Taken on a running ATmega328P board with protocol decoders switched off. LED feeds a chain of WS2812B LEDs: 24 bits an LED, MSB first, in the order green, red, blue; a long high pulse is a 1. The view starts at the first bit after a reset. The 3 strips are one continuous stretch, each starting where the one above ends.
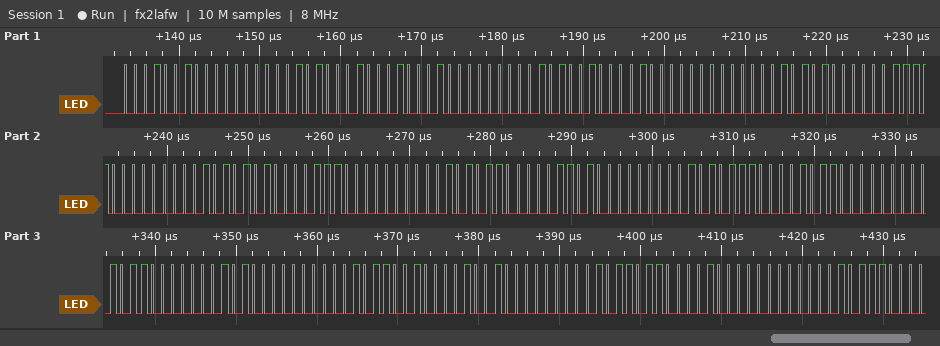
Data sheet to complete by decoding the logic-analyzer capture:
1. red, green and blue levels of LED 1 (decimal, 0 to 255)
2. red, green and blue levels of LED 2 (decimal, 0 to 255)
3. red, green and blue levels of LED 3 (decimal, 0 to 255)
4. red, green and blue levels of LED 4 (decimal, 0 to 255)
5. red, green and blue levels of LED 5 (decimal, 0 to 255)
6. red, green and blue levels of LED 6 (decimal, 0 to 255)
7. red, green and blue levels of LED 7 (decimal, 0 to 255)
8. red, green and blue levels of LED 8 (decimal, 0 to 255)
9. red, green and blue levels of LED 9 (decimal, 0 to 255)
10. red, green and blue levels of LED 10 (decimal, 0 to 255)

0, 18, 81
0, 17, 82
0, 16, 84
0, 15, 85
0, 14, 86
0, 13, 87
0, 11, 88
0, 10, 89
0, 9, 91
0, 8, 92
